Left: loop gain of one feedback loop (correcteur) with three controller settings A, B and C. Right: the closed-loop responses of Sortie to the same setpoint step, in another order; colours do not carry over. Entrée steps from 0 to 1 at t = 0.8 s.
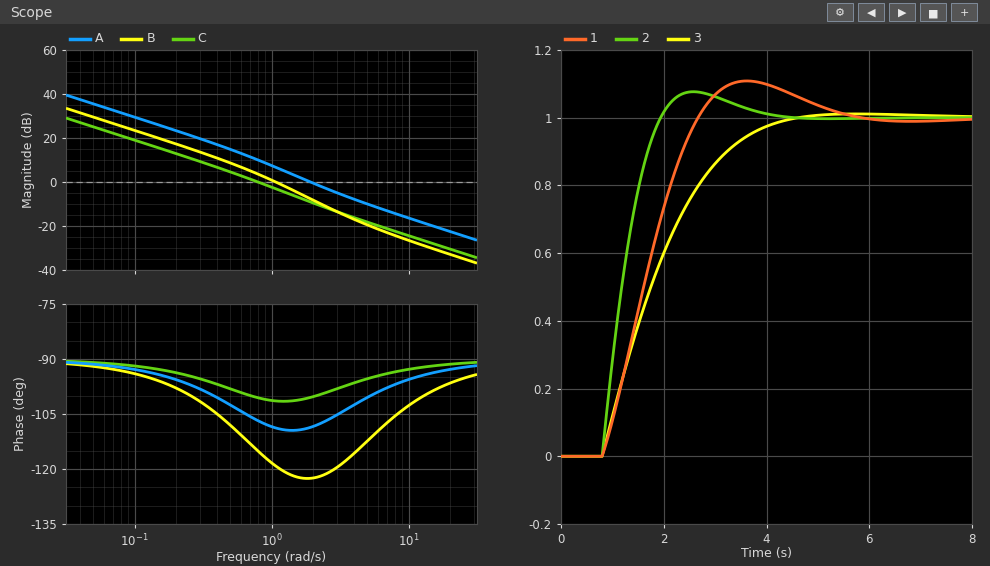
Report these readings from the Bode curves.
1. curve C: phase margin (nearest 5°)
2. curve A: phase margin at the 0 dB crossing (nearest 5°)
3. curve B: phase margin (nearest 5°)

80°
70°
60°
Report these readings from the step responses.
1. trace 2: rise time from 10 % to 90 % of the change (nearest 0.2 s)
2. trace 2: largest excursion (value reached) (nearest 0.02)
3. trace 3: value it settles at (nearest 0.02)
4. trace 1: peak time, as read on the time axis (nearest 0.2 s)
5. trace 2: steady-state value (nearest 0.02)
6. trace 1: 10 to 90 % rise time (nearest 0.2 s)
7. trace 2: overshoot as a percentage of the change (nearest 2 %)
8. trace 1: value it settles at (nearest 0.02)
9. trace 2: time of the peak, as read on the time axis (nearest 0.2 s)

0.8 s
1.08
1.00
3.6 s
1.00
1.4 s
8 %
1.00
2.6 s
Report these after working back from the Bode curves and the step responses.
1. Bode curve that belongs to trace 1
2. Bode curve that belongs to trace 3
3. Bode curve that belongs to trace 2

B
C
A
